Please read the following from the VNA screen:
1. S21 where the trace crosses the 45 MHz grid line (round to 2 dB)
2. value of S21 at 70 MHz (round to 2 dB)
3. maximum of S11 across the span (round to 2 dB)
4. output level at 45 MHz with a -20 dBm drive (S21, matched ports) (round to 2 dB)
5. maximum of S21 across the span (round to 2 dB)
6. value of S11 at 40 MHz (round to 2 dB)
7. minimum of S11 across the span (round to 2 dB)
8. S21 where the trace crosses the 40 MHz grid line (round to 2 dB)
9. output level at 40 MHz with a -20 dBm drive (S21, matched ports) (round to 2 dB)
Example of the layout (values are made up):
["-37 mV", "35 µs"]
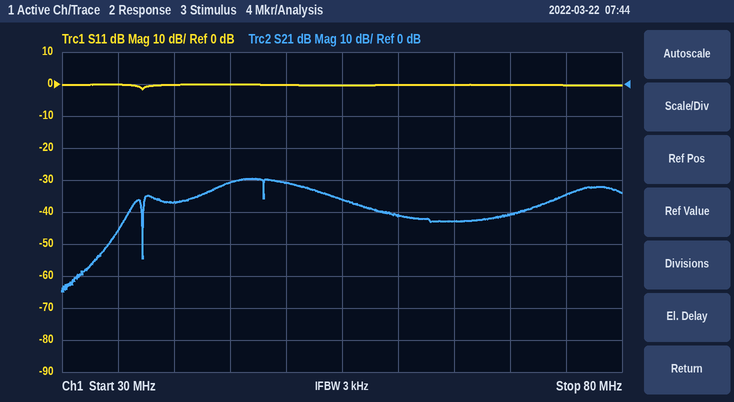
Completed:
["-30 dB", "-40 dB", "0 dB", "-50 dBm", "-30 dB", "0 dB", "-2 dB", "-36 dB", "-56 dBm"]
